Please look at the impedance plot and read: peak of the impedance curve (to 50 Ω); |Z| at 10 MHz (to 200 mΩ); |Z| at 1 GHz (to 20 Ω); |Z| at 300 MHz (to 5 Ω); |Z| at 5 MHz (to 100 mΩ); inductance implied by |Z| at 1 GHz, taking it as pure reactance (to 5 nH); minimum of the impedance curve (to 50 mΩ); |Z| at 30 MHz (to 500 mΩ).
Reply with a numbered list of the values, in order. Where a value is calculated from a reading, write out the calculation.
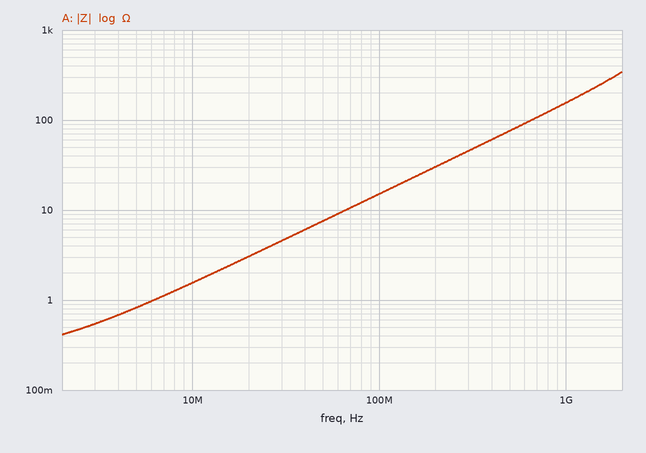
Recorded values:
1. 350 Ω
2. 1.6 Ω
3. 160 Ω
4. 45 Ω
5. 800 mΩ
6. L = 160 Ω/(2π × 1 GHz) ≈ 25 nH
7. 400 mΩ
8. 4.5 Ω
